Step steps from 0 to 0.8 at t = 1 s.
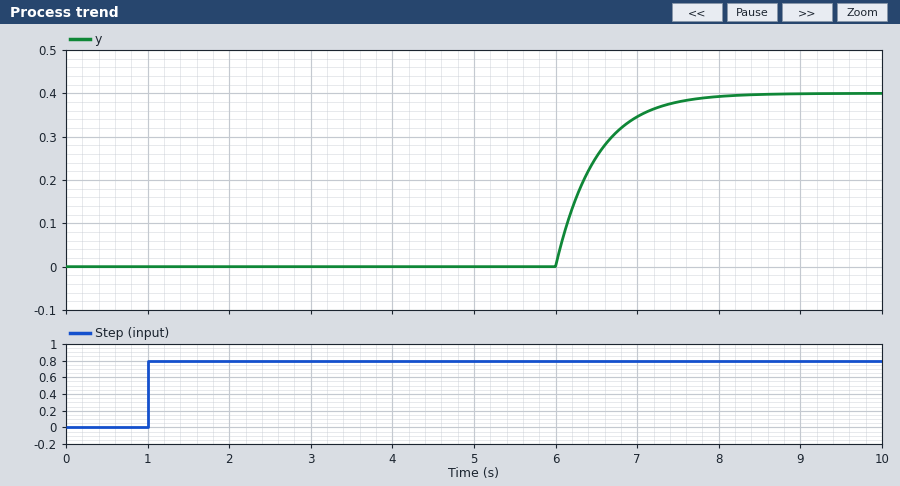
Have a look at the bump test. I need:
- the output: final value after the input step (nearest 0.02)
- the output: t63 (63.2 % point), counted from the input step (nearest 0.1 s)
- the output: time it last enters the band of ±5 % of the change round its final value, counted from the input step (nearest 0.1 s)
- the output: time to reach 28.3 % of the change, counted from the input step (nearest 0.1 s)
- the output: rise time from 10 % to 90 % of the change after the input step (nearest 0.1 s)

0.40
5.5 s
6.5 s
5.2 s
1.1 s
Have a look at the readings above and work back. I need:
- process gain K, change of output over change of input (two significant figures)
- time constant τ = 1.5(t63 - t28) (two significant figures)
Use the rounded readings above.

0.50
0.45 s
